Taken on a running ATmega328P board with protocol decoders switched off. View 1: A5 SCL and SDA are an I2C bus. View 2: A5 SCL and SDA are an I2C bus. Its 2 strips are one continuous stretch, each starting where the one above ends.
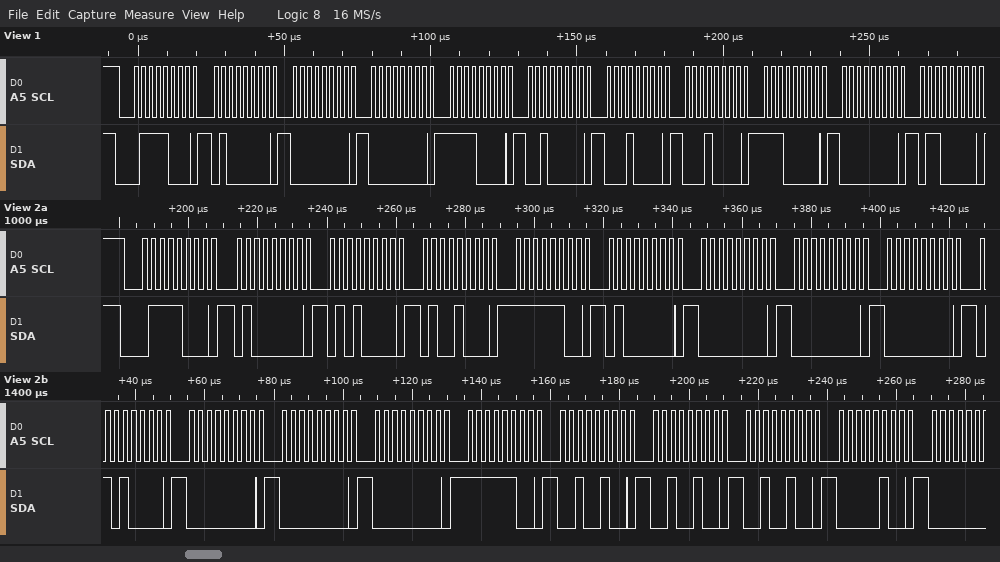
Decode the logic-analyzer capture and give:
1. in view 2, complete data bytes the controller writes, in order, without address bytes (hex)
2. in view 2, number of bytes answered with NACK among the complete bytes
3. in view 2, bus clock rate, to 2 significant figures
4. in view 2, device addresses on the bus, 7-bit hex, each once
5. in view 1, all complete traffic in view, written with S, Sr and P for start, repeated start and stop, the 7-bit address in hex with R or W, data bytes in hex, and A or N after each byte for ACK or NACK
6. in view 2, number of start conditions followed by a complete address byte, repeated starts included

40 50 48 FC 40 00 00 00 50 00 00 00 FC 24 24 24 04
0
400 kHz
0x3C
S 3CW A 40 A 00 A 00 A F0 A 20 A 10 A 10 A E0 A 00 A 60 A
1
